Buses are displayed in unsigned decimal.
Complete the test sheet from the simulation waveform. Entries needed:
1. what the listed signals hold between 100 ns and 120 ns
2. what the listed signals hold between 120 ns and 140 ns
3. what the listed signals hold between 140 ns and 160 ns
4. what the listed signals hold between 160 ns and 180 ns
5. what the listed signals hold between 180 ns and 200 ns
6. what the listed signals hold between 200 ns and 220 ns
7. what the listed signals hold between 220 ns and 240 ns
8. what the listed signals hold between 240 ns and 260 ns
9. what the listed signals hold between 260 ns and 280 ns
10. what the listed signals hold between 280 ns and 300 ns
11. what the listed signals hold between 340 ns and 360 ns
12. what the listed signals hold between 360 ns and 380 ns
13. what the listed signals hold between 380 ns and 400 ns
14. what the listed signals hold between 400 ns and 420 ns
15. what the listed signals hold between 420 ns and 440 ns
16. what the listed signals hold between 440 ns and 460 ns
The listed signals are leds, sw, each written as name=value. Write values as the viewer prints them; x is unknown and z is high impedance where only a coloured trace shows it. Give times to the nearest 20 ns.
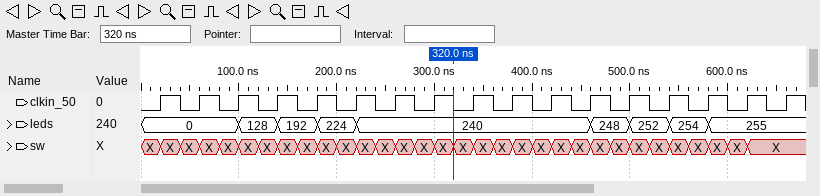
leds=128, sw=X
leds=128, sw=X
leds=192, sw=X
leds=192, sw=X
leds=224, sw=X
leds=224, sw=X
leds=240, sw=X
leds=240, sw=X
leds=240, sw=X
leds=240, sw=X
leds=240, sw=X
leds=240, sw=X
leds=240, sw=X
leds=240, sw=X
leds=240, sw=X
leds=240, sw=X
